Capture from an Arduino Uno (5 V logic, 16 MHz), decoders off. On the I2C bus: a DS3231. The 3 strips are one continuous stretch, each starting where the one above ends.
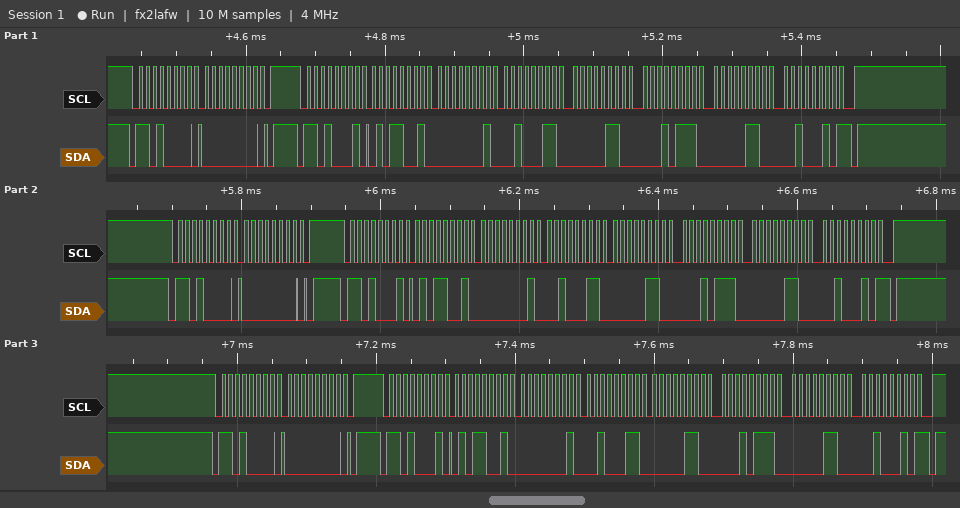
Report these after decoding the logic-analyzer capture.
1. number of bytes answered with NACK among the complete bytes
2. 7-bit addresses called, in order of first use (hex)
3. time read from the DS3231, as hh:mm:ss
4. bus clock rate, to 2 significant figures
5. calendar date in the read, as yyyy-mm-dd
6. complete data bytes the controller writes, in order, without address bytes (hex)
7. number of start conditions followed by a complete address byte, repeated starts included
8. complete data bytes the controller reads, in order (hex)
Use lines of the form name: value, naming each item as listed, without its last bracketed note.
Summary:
number of bytes answered with NACK among the complete bytes: 3
7-bit addresses called, in order of first use: 0x68
time read from the DS3231, as hh:mm:ss: 23:01:59
bus clock rate, to 2 significant figures: 100 kHz
calendar date in the read, as yyyy-mm-dd: 2022-06-17
complete data bytes the controller writes, in order, without address bytes: 00 00 00
number of start conditions followed by a complete address byte, repeated starts included: 6
complete data bytes the controller reads, in order: 59 01 23 06 17 06 22 59 01 23 06 17 06 22 59 01 23 06 17 06 22
